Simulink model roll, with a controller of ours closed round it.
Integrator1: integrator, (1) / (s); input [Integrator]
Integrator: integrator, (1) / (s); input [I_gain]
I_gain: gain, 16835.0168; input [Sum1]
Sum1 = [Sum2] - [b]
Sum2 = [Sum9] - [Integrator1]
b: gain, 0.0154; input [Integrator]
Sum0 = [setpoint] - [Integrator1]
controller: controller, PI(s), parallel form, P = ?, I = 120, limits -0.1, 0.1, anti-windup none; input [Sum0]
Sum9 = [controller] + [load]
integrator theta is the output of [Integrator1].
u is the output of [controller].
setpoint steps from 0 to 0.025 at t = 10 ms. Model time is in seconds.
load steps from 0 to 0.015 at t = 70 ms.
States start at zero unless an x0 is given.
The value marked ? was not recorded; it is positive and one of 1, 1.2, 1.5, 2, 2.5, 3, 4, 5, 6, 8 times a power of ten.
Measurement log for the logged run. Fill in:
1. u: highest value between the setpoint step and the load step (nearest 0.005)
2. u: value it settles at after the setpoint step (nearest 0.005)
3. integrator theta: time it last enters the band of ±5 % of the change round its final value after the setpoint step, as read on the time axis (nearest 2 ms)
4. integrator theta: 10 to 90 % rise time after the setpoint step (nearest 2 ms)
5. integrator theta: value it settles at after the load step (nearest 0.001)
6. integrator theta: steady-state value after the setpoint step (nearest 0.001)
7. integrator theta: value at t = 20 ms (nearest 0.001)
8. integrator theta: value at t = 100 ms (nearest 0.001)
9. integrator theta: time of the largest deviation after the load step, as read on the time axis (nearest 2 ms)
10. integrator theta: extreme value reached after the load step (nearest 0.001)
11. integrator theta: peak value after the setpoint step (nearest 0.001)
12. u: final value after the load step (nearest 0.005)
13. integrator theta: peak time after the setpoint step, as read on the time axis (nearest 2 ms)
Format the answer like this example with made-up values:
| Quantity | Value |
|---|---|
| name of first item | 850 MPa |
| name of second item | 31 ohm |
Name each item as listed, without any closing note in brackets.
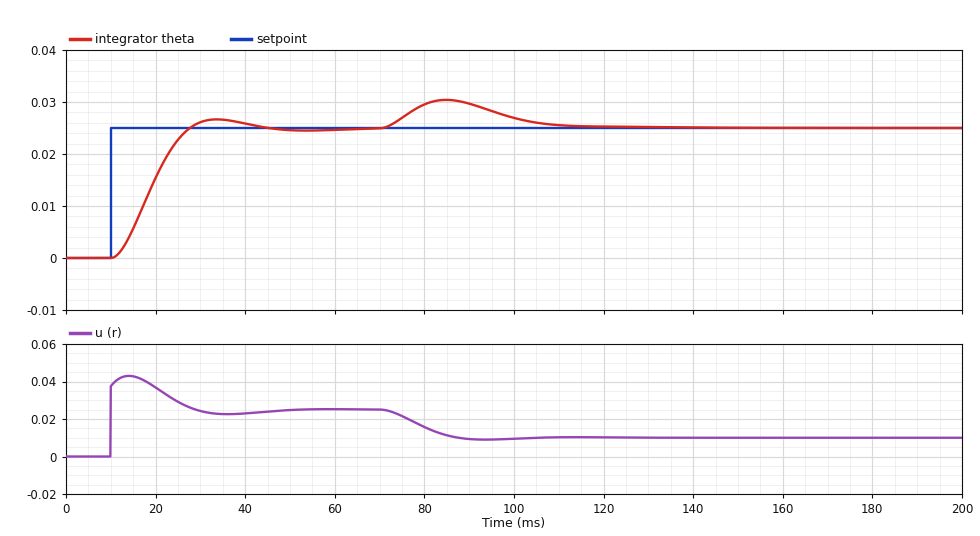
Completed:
| Quantity | Value |
|---|---|
| u: highest value between the setpoint step and the load step | 0.045 |
| u: value it settles at after the setpoint step | 0.025 |
| integrator theta: time it last enters the band of ±5 % of the change round its final value after the setpoint step, as read on the time axis | 38 ms |
| integrator theta: 10 to 90 % rise time after the setpoint step | 12 ms |
| integrator theta: value it settles at after the load step | 0.025 |
| integrator theta: steady-state value after the setpoint step | 0.025 |
| integrator theta: value at t = 20 ms | 0.015 |
| integrator theta: value at t = 100 ms | 0.027 |
| integrator theta: time of the largest deviation after the load step, as read on the time axis | 84 ms |
| integrator theta: extreme value reached after the load step | 0.030 |
| integrator theta: peak value after the setpoint step | 0.027 |
| u: final value after the load step | 0.010 |
| integrator theta: peak time after the setpoint step, as read on the time axis | 34 ms |
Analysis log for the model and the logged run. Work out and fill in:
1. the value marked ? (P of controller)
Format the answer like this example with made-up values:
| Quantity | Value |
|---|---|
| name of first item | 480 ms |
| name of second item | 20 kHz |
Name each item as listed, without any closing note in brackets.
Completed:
| Quantity | Value |
|---|---|
| the value marked ? | 1.5 |
